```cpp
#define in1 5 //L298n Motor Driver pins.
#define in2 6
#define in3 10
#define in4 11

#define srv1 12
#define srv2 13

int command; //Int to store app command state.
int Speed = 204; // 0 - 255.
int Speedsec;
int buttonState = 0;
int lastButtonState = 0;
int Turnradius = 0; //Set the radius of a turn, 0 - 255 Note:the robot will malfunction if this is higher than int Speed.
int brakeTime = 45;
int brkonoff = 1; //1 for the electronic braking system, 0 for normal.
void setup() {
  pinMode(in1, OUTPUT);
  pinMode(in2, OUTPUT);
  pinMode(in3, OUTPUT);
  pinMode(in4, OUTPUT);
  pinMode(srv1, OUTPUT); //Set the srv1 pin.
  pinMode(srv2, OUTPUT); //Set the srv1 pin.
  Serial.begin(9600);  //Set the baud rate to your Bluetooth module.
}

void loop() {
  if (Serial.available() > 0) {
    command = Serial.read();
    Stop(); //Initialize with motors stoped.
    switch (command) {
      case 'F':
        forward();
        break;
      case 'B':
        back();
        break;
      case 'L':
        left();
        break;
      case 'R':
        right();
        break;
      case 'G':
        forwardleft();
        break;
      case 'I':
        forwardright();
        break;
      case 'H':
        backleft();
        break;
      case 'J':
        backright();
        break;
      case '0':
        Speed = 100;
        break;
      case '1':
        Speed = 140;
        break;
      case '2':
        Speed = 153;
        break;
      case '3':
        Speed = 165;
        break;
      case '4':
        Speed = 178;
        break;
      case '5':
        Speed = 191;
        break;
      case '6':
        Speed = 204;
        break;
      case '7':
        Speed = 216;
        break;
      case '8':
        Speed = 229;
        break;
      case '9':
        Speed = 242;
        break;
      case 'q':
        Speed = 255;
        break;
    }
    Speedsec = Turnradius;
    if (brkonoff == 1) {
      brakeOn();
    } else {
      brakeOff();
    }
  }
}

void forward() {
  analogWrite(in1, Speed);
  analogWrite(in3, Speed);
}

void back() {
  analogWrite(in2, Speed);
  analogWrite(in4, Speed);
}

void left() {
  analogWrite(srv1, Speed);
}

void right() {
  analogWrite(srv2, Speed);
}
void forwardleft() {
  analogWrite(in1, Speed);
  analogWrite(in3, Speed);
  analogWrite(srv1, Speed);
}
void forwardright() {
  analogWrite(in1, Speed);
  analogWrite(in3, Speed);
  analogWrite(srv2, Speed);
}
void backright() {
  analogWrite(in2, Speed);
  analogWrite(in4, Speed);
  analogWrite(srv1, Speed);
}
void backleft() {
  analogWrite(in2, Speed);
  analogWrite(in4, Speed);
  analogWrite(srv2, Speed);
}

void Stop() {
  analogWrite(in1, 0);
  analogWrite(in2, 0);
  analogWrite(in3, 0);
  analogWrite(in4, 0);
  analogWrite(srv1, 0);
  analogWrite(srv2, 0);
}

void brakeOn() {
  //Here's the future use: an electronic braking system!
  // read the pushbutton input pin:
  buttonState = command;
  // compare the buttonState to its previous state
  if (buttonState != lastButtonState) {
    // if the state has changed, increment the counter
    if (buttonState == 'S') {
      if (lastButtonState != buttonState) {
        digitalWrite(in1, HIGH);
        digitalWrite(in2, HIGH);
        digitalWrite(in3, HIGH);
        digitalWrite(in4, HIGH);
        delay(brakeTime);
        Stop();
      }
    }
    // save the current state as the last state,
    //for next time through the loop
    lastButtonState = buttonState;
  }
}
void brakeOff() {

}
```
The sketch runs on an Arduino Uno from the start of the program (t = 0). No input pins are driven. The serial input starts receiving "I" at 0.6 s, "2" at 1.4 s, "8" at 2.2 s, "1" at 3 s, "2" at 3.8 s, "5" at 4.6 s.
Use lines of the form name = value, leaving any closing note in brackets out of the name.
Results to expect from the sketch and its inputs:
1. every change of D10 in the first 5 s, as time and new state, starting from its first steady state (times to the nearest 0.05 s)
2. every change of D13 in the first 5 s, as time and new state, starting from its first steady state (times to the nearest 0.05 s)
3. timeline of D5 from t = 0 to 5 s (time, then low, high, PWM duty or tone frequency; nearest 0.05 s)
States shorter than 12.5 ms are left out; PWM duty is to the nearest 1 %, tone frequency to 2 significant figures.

every change of D10 in the first 5 s, as time and new state, starting from its first steady state = 0 s low; 0.6 s PWM 80 %; 1.4 s low
every change of D13 in the first 5 s, as time and new state, starting from its first steady state = 0 s low; 0.6 s high; 1.4 s low
timeline of D5 from t = 0 to 5 s = 0 s low; 0.6 s PWM 80 %; 1.4 s low
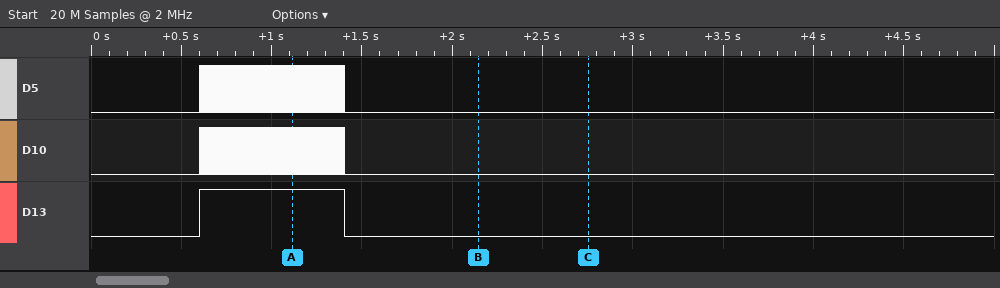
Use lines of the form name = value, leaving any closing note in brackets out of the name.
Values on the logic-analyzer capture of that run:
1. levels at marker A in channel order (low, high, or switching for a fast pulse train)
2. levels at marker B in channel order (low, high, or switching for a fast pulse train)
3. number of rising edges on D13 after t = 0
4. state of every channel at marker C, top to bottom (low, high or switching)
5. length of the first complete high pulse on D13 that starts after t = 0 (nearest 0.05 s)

levels at marker A in channel order = D5 switching, D10 switching, D13 high
levels at marker B in channel order = D5 low, D10 low, D13 low
number of rising edges on D13 after t = 0 = 1
state of every channel at marker C, top to bottom = D5 low, D10 low, D13 low
length of the first complete high pulse on D13 that starts after t = 0 = 0.80 s
